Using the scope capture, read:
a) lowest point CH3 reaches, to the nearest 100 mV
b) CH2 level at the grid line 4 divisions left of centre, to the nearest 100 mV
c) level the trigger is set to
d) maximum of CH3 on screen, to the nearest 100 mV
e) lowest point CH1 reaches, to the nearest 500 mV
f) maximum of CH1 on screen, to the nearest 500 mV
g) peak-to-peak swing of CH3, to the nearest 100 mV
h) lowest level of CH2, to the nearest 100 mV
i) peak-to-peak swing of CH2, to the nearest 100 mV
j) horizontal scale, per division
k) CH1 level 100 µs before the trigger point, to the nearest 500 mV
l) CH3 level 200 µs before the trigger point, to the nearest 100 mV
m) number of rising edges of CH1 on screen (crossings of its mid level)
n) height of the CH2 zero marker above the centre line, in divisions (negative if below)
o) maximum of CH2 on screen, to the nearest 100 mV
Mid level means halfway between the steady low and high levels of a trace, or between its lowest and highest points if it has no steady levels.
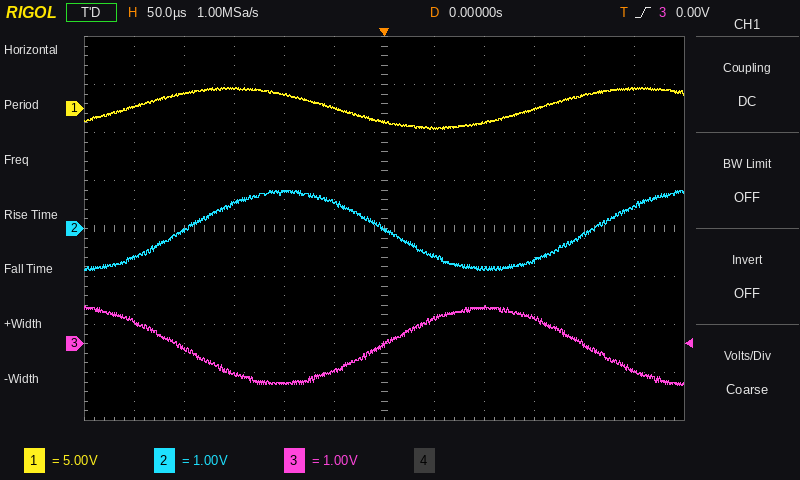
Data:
-900 mV
0.0 V
0.00 V
800 mV
-2.0 V
2.0 V
1.7 V
-900 mV
1.7 V
50 µs
1.5 V
-100 mV
2
0.0 div
800 mV
